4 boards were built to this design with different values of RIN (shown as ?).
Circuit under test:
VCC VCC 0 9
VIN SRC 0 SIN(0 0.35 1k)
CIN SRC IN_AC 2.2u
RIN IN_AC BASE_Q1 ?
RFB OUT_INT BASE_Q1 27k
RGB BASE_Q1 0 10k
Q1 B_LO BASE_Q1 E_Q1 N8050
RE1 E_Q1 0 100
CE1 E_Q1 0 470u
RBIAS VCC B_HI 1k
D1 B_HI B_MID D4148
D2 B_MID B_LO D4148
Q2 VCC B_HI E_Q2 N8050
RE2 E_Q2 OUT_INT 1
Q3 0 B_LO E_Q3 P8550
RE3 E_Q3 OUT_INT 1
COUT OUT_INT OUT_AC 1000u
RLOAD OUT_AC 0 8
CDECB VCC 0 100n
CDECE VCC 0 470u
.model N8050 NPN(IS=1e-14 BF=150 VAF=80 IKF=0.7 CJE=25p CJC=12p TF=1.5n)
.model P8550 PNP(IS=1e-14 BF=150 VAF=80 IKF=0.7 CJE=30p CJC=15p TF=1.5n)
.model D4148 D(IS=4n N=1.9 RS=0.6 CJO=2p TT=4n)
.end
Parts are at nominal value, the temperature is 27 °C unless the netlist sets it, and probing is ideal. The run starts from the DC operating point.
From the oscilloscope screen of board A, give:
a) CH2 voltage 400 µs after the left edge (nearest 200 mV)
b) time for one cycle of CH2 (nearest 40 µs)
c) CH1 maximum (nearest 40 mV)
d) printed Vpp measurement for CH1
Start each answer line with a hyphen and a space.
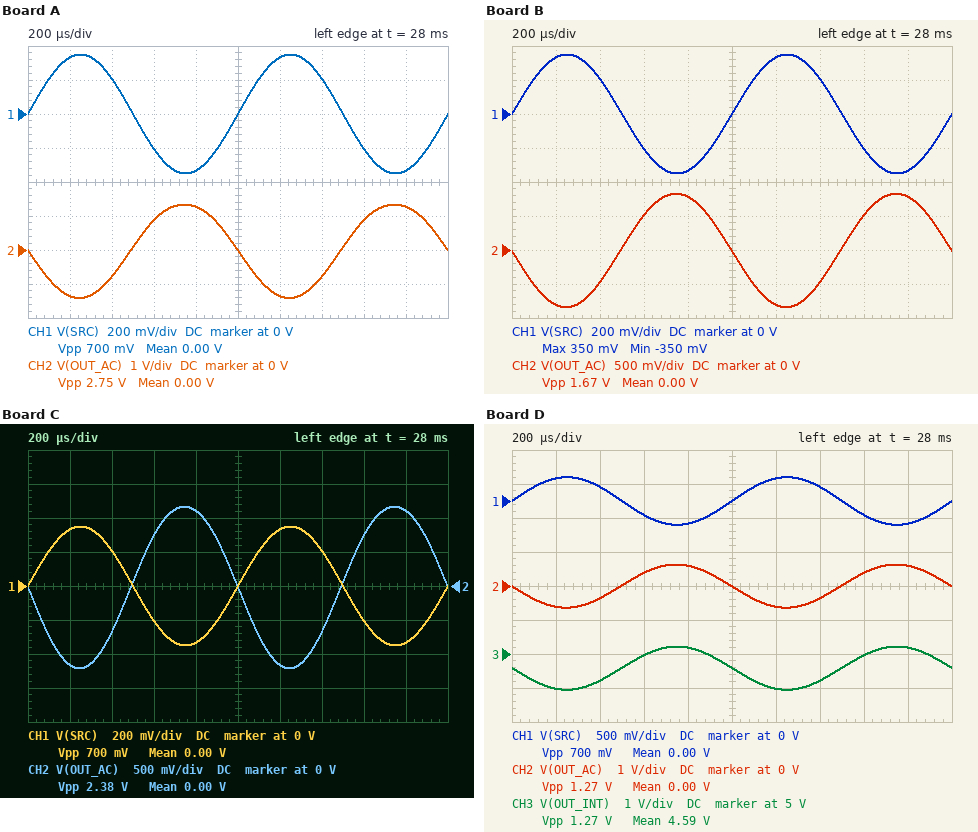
- -800 mV
- 1.00 ms
- 360 mV
- 700 mV
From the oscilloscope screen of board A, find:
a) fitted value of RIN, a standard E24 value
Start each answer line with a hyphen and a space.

- 4.3 kΩ
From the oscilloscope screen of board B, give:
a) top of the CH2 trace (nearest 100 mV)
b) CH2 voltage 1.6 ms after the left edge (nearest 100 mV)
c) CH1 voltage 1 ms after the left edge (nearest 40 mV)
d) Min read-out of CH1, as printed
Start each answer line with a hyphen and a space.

- 800 mV
- 500 mV
- 0 V
- -350 mV
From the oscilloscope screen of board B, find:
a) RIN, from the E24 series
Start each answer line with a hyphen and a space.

- 7.5 kΩ
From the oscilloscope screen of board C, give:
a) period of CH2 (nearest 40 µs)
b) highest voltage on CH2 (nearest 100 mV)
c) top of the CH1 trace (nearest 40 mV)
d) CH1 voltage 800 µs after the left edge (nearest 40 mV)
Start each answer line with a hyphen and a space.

- 1.00 ms
- 1.2 V
- 360 mV
- -320 mV
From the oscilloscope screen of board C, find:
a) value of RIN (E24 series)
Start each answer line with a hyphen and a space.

- 5.1 kΩ
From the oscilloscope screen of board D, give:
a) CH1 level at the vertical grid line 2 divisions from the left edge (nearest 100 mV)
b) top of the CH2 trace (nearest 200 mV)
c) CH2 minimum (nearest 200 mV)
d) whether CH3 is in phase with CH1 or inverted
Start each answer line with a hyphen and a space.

- 200 mV
- 600 mV
- -600 mV
- inverted
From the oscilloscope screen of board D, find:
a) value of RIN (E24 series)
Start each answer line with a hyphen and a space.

- 10 kΩ
